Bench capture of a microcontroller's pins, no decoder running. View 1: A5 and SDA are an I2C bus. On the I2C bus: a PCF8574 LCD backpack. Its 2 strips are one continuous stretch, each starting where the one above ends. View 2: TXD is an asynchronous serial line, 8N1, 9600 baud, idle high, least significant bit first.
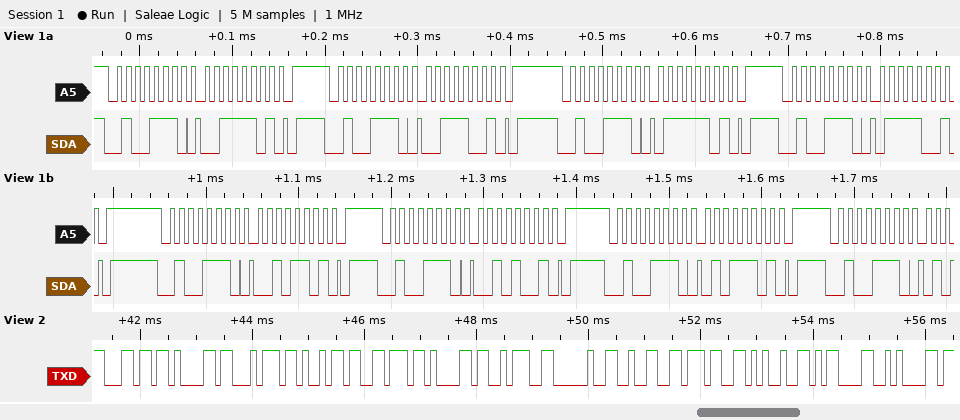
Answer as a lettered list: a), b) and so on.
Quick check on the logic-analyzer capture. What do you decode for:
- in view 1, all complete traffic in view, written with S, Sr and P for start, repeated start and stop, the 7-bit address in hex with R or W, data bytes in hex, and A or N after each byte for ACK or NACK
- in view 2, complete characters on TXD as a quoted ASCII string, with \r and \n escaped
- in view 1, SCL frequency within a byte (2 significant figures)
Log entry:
a) S 27W A 3D A P S 27W A 39 A P S 27W A 7D A P S 27W A 79 A P S 27W A 2D A P S 27W A 29 A P S 27W A 5D A P S 27W A
b) "lativa: 27%\r\n"
c) 100 kHz
